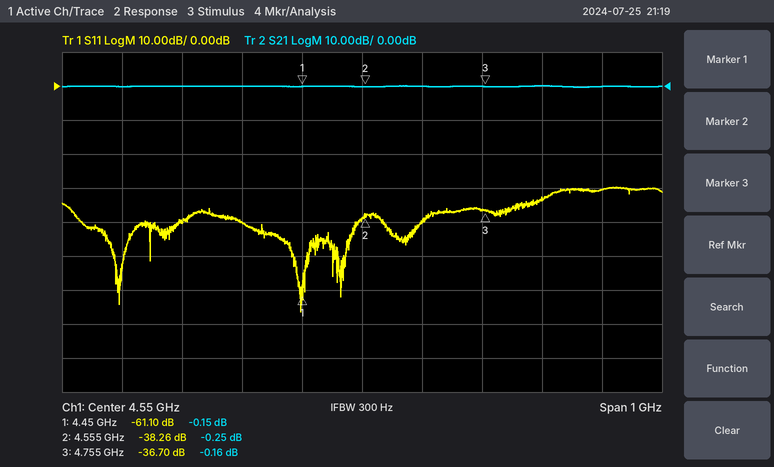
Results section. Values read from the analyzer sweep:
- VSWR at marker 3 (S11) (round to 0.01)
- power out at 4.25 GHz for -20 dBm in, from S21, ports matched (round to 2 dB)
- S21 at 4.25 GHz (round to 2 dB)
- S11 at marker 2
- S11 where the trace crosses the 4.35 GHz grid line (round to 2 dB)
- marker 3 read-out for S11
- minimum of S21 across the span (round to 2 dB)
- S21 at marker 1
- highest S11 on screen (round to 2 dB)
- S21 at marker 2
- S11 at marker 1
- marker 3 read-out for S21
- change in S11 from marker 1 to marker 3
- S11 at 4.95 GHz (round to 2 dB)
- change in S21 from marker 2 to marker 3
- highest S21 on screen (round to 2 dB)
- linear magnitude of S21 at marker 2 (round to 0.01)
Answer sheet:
1.03
-20 dBm
0 dB
-38.26 dB
-40 dB
-36.70 dB
0 dB
-0.15 dB
-30 dB
-0.25 dB
-61.10 dB
-0.16 dB
24.40 dB
-30 dB
0.09 dB
0 dB
0.97
